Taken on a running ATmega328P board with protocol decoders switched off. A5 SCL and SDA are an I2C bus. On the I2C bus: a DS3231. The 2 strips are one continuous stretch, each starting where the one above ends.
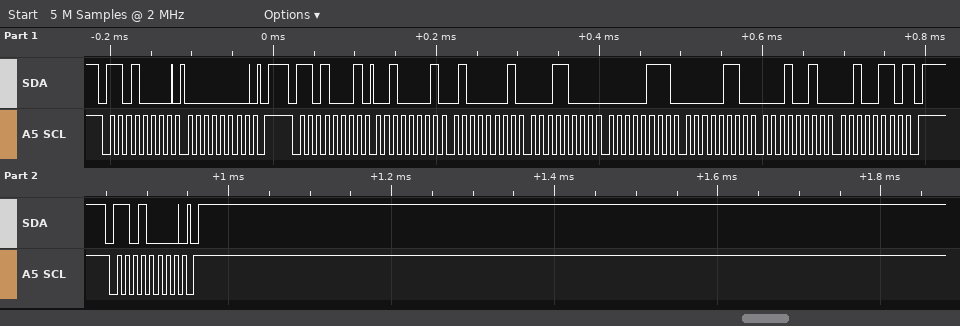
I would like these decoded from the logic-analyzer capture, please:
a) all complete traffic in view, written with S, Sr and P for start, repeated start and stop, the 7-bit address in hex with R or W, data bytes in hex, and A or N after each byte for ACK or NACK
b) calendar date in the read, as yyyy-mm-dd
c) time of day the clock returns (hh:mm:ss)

S 68W A 00 A P S 68R A 21 A 41 A 18 A 07 A 06 A 12 A 26 N P S 68W A P
2026-12-06
18:41:21
